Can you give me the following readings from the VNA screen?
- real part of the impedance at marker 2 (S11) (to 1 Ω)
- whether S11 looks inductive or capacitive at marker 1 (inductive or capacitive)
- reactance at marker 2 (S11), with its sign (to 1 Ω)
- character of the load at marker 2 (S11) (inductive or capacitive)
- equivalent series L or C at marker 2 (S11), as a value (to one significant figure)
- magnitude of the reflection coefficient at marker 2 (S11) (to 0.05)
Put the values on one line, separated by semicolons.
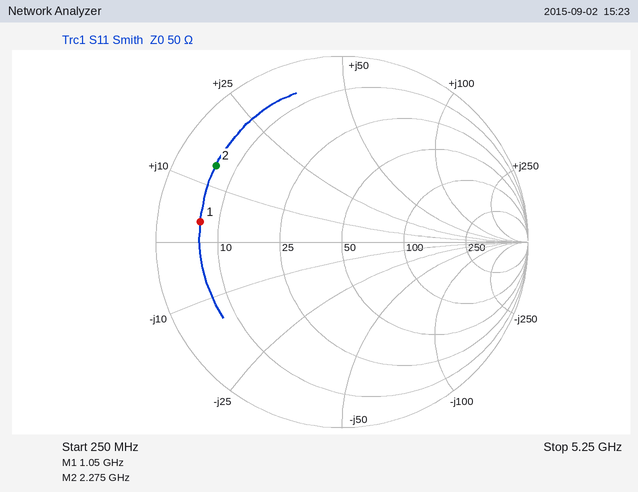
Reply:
6 Ω; inductive; +14 Ω; inductive; 1.0 nH; 0.80
